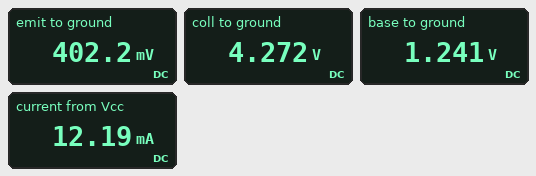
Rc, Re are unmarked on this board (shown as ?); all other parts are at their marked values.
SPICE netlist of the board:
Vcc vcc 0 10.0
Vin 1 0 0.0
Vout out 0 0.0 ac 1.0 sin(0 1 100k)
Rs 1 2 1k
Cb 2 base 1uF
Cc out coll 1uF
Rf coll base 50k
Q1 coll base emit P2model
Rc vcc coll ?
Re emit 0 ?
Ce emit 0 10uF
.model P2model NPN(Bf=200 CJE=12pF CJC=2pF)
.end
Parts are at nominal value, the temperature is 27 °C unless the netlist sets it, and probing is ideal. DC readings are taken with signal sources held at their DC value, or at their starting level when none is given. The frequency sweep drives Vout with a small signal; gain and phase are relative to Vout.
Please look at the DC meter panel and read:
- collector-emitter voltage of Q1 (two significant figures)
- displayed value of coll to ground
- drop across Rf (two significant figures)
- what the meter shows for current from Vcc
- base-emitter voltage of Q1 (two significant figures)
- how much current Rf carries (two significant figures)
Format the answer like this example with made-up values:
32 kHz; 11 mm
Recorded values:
3.9 V; 4.272 V; 3.0 V; 12.19 mA; 840 mV; 61 µA
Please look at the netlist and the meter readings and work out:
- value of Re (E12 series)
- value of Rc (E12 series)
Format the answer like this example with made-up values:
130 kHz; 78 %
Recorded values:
33 Ω; 470 Ω
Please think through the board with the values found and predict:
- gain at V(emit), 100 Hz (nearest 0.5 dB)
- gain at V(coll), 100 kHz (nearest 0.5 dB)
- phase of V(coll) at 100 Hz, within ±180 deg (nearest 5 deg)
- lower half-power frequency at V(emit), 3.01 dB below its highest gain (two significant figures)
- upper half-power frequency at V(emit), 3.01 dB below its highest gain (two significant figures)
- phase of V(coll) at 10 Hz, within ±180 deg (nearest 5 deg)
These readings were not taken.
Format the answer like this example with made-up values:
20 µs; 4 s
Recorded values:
-44.0 dB; 0 dB; 90 deg; 230 Hz; 3.8 kHz; 100 deg
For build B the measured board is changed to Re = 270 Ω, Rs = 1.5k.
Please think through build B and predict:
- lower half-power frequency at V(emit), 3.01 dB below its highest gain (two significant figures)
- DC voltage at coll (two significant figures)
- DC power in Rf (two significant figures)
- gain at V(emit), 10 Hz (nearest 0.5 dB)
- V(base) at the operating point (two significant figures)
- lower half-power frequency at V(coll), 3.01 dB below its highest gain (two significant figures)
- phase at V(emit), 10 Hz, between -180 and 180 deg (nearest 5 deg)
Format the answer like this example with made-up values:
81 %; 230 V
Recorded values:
200 Hz; 5.6 V; 110 µW; -45.0 dB; 3.3 V; 590 Hz; 45 deg
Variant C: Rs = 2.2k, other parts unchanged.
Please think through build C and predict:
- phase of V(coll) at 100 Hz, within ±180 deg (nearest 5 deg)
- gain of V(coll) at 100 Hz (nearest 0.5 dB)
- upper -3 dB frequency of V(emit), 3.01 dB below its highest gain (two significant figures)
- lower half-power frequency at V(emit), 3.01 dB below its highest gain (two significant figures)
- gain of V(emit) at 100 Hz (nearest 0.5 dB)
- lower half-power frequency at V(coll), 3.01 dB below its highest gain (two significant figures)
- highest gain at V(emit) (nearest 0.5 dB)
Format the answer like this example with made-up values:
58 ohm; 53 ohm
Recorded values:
85 deg; -14.0 dB; 2.9 kHz; 280 Hz; -43.0 dB; 680 Hz; -34.0 dB
